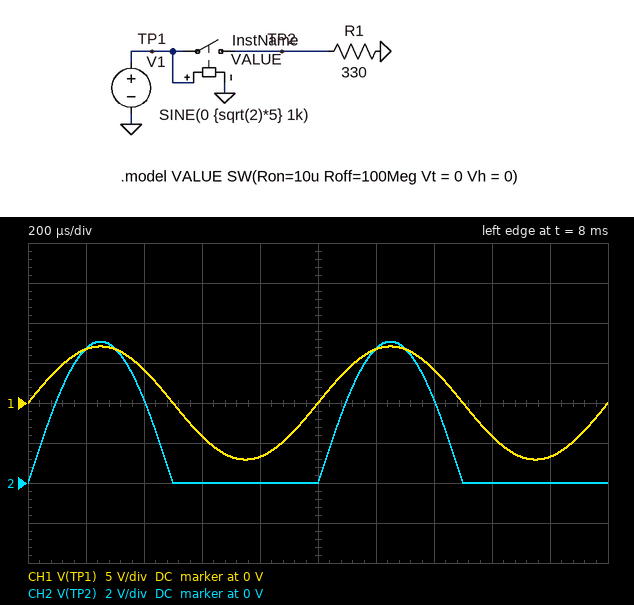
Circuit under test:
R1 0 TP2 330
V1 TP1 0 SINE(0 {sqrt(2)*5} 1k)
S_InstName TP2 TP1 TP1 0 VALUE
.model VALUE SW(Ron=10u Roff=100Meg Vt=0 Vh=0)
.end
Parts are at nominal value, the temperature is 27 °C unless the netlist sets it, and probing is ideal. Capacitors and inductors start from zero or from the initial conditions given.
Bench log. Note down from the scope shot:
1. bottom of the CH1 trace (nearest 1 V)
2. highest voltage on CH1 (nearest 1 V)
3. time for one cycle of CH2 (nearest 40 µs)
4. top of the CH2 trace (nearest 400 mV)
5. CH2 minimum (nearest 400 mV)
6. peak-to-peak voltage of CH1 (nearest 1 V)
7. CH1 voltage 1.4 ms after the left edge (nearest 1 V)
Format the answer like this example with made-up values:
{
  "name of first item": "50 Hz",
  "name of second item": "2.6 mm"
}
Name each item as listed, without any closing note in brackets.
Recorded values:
{
  "bottom of the CH1 trace": "-7 V",
  "highest voltage on CH1": "7 V",
  "time for one cycle of CH2": "1.00 ms",
  "top of the CH2 trace": "7.2 V",
  "CH2 minimum": "0 V",
  "peak-to-peak voltage of CH1": "14 V",
  "CH1 voltage 1.4 ms after the left edge": "4 V"
}
